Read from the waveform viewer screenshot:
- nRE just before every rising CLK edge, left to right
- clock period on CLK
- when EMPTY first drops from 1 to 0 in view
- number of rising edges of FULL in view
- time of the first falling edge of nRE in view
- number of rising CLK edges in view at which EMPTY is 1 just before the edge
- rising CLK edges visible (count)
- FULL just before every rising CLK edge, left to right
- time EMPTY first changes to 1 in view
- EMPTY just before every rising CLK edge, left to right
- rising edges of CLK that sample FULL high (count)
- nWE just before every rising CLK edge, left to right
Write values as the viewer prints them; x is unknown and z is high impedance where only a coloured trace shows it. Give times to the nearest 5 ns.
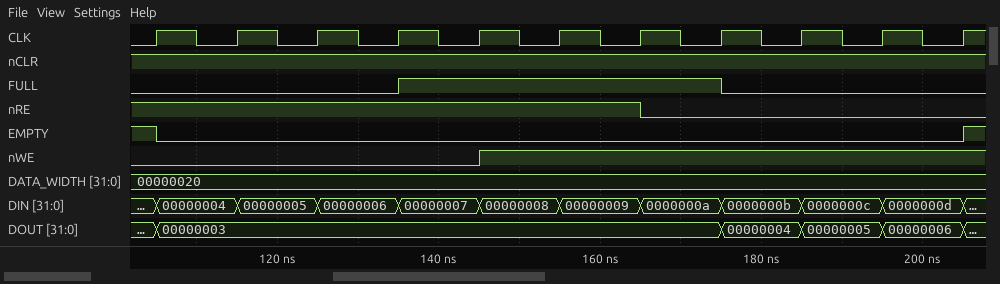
1 1 1 1 1 1 1 0 0 0 0
10 ns
105 ns
1
165 ns
1
11
0 0 0 0 1 1 1 1 0 0 0
205 ns
1 0 0 0 0 0 0 0 0 0 0
4
0 0 0 0 0 1 1 1 1 1 1
